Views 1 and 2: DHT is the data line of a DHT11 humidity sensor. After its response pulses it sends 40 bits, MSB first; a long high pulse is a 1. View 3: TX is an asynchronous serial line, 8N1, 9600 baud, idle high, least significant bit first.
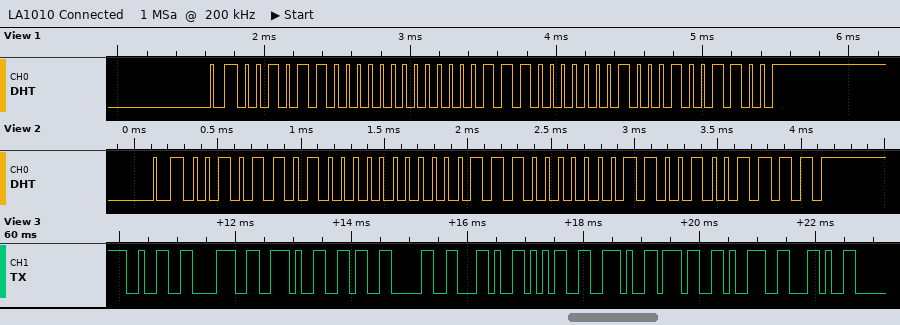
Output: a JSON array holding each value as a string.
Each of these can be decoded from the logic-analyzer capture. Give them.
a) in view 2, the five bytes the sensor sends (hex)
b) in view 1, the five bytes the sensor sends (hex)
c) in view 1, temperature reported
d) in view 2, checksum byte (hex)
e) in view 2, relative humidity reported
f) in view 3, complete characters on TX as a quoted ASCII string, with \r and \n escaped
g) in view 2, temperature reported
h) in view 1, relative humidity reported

["2D 00 1C 06 4F", "2C 00 1C 04 4C", "28.4 °C", "0x4F", "45 %", "\"28.60,5.79,\"", "28.6 °C", "44 %"]
